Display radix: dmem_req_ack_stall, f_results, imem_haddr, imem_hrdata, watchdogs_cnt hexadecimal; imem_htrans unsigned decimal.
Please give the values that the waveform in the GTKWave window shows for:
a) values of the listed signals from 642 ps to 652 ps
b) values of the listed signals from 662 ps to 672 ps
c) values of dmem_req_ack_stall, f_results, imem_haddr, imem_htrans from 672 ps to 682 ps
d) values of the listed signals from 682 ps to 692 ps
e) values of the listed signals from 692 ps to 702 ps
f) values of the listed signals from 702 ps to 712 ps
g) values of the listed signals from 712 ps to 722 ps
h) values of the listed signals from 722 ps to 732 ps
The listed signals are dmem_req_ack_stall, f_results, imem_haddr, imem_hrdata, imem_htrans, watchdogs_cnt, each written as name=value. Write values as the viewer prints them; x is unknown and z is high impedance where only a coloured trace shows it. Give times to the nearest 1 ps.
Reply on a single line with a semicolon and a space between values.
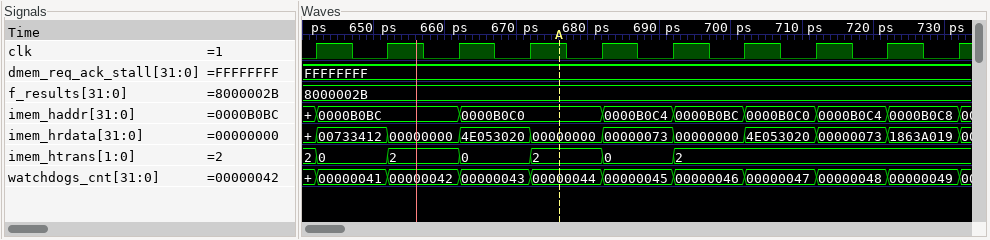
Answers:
dmem_req_ack_stall=FFFFFFFF, f_results=8000002B, imem_haddr=0000B0BC, imem_hrdata=00733412, imem_htrans=0, watchdogs_cnt=00000041; dmem_req_ack_stall=FFFFFFFF, f_results=8000002B, imem_haddr=0000B0C0, imem_hrdata=4E053020, imem_htrans=0, watchdogs_cnt=00000043; dmem_req_ack_stall=FFFFFFFF, f_results=8000002B, imem_haddr=0000B0C0, imem_htrans=2; dmem_req_ack_stall=FFFFFFFF, f_results=8000002B, imem_haddr=0000B0C4, imem_hrdata=00000073, imem_htrans=0, watchdogs_cnt=00000045; dmem_req_ack_stall=FFFFFFFF, f_results=8000002B, imem_haddr=0000B0BC, imem_hrdata=00000000, imem_htrans=2, watchdogs_cnt=00000046; dmem_req_ack_stall=FFFFFFFF, f_results=8000002B, imem_haddr=0000B0C0, imem_hrdata=4E053020, imem_htrans=2, watchdogs_cnt=00000047; dmem_req_ack_stall=FFFFFFFF, f_results=8000002B, imem_haddr=0000B0C4, imem_hrdata=00000073, imem_htrans=2, watchdogs_cnt=00000048; dmem_req_ack_stall=FFFFFFFF, f_results=8000002B, imem_haddr=0000B0C8, imem_hrdata=1863A019, imem_htrans=2, watchdogs_cnt=00000049
